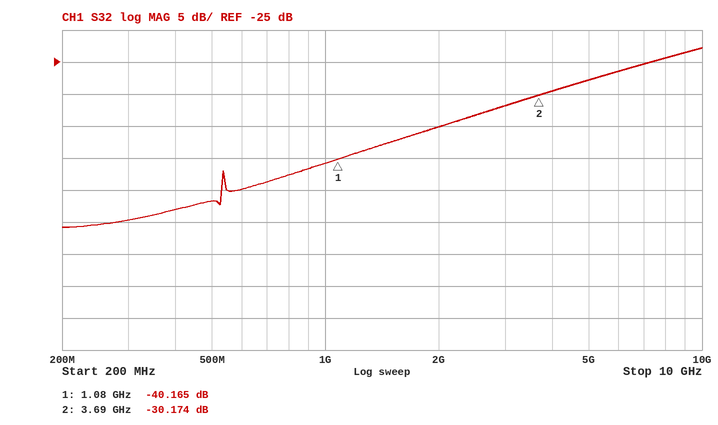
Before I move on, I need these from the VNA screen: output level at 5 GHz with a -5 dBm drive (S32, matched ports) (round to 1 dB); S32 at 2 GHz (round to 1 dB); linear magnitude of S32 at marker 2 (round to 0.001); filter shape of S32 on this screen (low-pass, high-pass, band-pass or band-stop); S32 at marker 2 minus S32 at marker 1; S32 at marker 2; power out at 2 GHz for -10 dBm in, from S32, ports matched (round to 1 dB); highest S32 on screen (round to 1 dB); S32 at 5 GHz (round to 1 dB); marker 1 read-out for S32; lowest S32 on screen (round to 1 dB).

-33 dBm
-35 dB
0.031
high-pass
9.991 dB
-30.174 dB
-45 dBm
-23 dB
-28 dB
-40.165 dB
-51 dB
